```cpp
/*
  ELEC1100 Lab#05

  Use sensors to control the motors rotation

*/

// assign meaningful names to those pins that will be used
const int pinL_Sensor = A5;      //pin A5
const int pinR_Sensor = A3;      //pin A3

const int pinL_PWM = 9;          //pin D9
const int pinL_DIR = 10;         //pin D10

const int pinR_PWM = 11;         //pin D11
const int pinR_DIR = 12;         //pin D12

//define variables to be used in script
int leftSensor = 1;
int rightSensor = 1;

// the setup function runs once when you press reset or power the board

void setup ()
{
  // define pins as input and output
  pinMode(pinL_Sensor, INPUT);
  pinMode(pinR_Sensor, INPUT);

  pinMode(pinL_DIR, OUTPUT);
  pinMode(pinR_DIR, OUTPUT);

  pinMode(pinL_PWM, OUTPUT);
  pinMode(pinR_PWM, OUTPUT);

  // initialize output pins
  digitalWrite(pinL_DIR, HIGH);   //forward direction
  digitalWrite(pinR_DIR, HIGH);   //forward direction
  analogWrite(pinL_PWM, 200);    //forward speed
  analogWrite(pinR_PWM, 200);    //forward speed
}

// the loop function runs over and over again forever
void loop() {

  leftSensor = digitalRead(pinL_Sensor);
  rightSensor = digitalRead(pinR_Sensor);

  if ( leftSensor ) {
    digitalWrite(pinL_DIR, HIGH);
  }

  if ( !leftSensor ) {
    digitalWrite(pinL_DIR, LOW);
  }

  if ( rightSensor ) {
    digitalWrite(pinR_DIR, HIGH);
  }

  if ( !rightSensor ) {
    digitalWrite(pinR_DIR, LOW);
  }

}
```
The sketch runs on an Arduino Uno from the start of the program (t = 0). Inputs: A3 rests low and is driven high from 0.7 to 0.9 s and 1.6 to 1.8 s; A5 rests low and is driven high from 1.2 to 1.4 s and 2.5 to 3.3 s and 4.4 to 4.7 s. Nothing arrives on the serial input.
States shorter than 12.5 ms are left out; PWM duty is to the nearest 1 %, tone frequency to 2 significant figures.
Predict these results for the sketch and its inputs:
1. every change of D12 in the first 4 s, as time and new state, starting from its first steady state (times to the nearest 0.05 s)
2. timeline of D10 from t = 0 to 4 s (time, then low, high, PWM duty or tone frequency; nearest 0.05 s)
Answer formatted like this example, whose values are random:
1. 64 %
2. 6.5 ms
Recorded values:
1. 0 s low; 0.7 s high; 0.9 s low; 1.6 s high; 1.8 s low
2. 0 s low; 1.2 s high; 1.4 s low; 2.5 s high; 3.3 s low
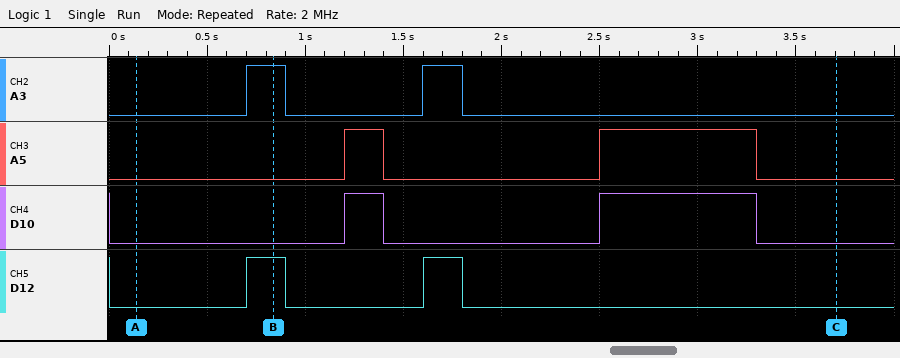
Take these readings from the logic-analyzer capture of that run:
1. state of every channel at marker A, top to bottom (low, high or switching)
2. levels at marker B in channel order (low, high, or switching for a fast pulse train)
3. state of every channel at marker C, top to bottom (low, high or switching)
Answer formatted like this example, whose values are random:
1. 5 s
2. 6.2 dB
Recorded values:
1. A3 low, A5 low, D10 low, D12 low
2. A3 high, A5 low, D10 low, D12 high
3. A3 low, A5 low, D10 low, D12 low
